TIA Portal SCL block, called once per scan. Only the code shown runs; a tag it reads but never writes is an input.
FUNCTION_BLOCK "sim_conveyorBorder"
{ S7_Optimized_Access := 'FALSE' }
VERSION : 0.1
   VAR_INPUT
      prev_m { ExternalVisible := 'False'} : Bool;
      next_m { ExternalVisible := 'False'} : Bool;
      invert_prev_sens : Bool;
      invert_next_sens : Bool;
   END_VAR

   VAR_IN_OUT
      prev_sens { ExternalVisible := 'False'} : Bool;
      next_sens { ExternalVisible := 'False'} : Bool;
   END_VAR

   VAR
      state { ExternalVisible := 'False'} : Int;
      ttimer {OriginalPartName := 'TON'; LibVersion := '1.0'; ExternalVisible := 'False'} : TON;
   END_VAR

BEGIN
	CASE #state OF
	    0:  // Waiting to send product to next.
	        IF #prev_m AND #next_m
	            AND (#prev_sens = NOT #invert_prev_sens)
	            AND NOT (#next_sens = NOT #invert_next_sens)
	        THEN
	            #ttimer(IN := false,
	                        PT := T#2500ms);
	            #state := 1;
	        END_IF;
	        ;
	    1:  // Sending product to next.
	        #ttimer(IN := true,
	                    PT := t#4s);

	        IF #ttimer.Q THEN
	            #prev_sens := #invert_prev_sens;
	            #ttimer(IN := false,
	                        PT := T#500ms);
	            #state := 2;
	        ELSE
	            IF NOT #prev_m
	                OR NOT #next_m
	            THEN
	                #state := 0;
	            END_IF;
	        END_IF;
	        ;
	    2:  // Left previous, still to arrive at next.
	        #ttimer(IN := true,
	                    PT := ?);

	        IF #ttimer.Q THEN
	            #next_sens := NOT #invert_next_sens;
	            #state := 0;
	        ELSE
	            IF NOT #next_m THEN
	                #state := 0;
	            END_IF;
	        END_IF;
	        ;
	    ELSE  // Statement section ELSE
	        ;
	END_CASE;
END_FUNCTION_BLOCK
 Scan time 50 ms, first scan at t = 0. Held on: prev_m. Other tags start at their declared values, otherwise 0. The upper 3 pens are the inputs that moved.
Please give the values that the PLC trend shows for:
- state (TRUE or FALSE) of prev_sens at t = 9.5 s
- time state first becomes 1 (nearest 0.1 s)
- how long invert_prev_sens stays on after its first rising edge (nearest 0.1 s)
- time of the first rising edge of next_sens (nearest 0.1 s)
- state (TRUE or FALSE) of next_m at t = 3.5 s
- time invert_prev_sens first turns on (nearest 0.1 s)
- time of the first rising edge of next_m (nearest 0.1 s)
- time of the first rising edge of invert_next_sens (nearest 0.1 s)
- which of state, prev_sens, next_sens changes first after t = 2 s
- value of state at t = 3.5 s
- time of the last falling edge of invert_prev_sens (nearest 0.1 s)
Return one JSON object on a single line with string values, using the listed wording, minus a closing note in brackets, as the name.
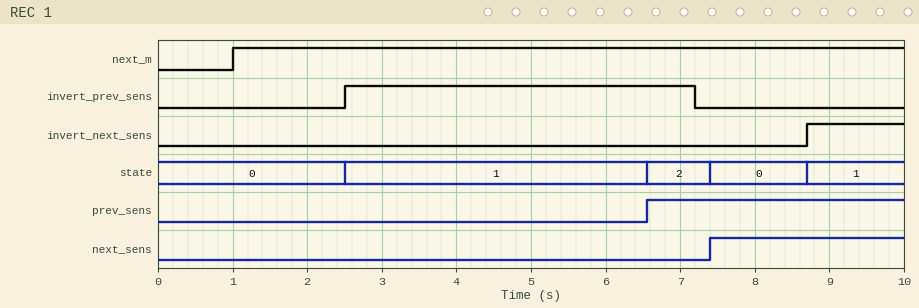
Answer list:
{"state (TRUE or FALSE) of prev_sens at t = 9.5 s": "TRUE", "time state first becomes 1": "2.5 s", "how long invert_prev_sens stays on after its first rising edge": "4.7 s", "time of the first rising edge of next_sens": "7.4 s", "state (TRUE or FALSE) of next_m at t = 3.5 s": "TRUE", "time invert_prev_sens first turns on": "2.5 s", "time of the first rising edge of next_m": "1.0 s", "time of the first rising edge of invert_next_sens": "8.7 s", "which of state, prev_sens, next_sens changes first after t = 2 s": "state", "value of state at t = 3.5 s": "1", "time of the last falling edge of invert_prev_sens": "7.2 s"}
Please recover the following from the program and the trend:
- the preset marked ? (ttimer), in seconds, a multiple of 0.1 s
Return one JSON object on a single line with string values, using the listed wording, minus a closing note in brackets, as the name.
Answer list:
{"the preset marked ? (ttimer), in seconds, a multiple of 0.1 s": "0.8 s"}
